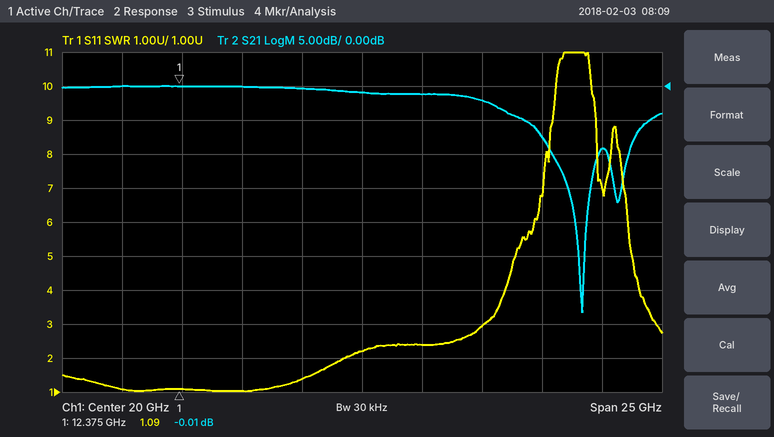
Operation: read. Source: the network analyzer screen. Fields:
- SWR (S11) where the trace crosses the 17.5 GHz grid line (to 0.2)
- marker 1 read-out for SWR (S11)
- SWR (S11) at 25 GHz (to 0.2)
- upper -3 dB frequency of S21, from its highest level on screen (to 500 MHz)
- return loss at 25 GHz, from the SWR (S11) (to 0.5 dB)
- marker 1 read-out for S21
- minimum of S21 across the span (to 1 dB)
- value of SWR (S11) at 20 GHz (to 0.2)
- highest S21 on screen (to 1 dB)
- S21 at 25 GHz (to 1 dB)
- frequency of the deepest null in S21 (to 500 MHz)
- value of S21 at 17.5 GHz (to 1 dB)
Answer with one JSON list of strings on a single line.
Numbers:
["1.4", "1.09", "3.0", "25.5 GHz", "6.0 dB", "-0.01 dB", "-33 dB", "2.2", "0 dB", "-2 dB", "29.0 GHz", "0 dB"]
